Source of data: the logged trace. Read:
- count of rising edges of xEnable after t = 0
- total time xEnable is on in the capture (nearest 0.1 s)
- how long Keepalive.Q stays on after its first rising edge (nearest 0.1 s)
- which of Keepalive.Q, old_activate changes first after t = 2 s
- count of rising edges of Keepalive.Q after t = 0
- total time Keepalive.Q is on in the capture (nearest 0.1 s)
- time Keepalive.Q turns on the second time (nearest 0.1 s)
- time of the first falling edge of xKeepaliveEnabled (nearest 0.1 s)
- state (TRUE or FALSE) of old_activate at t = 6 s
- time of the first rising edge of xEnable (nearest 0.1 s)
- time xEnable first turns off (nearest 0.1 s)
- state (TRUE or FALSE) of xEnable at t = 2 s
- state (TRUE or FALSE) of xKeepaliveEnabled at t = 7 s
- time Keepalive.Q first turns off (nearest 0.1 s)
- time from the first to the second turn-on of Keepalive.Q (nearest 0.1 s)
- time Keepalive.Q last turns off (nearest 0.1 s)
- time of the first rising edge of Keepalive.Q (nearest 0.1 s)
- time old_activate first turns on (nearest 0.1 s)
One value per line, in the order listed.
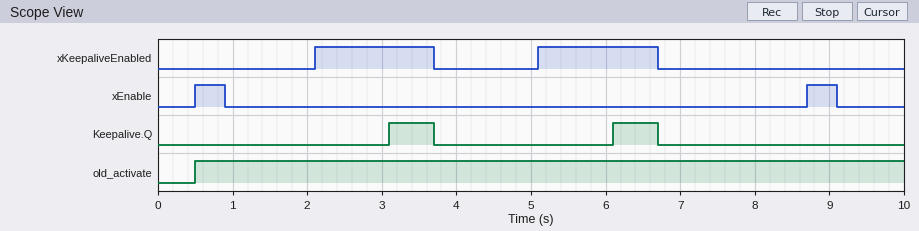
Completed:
2
0.8 s
0.6 s
Keepalive.Q
2
1.2 s
6.1 s
3.7 s
TRUE
0.5 s
0.9 s
FALSE
FALSE
3.7 s
3.0 s
6.7 s
3.1 s
0.5 s
